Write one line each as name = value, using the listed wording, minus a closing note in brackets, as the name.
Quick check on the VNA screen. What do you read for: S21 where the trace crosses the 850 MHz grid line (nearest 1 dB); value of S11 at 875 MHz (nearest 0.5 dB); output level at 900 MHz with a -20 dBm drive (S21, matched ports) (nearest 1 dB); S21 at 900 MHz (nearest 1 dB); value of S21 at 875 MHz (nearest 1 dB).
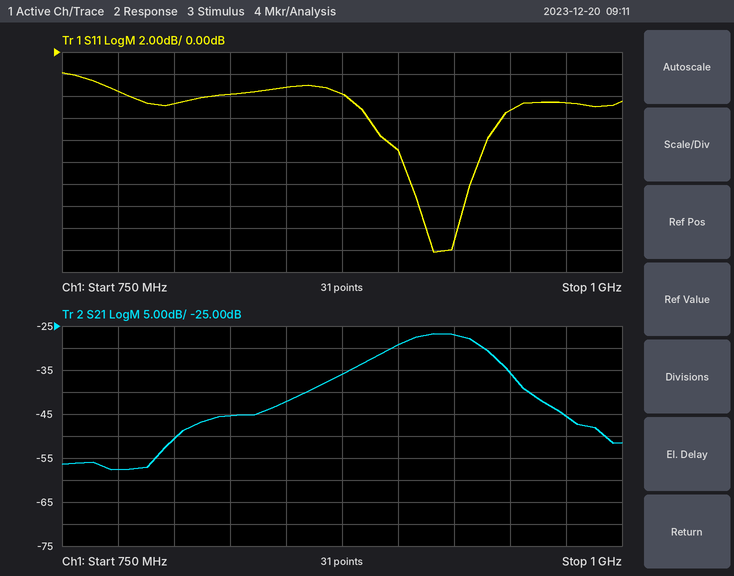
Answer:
S21 where the trace crosses the 850 MHz grid line = -42 dB
value of S11 at 875 MHz = -4.0 dB
output level at 900 MHz with a -20 dBm drive (S21, matched ports) = -49 dBm
S21 at 900 MHz = -29 dB
value of S21 at 875 MHz = -36 dB
